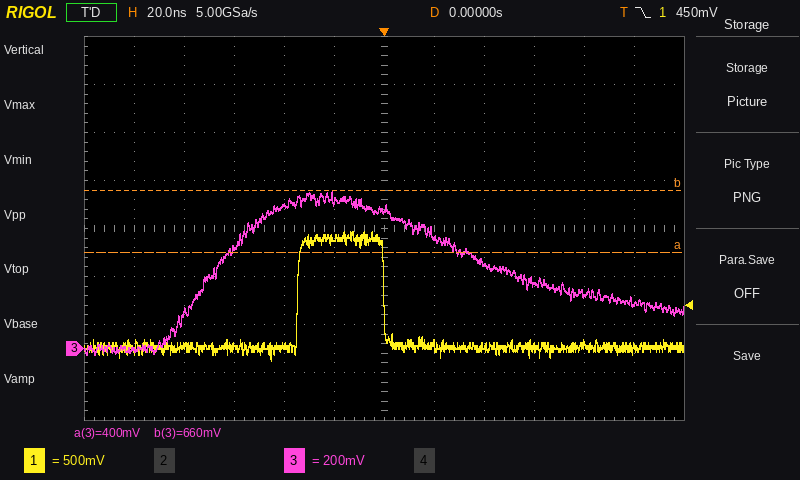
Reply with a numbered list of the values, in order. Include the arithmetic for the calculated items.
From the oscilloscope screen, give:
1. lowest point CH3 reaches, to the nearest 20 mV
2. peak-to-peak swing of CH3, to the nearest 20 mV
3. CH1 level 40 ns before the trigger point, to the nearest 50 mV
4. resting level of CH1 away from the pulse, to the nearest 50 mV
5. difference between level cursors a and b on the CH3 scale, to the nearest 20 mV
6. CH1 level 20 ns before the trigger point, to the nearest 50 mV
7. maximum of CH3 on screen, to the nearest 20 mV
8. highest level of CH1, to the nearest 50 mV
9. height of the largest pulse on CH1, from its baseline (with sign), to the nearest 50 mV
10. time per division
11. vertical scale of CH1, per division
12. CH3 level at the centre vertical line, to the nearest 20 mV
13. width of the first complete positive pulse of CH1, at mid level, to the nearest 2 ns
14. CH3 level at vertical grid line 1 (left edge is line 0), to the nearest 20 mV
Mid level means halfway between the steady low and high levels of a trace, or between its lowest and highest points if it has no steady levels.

1. -20 mV
2. 660 mV − (-20 mV) = 680 mV
3. 50 mV
4. 0 mV
5. 260 mV
6. 1.15 V
7. 660 mV
8. 1.20 V
9. 1.20 V − (0 mV) = +1.20 V
10. 20 ns
11. 500 mV
12. 580 mV
13. 34 ns
14. 0 mV
